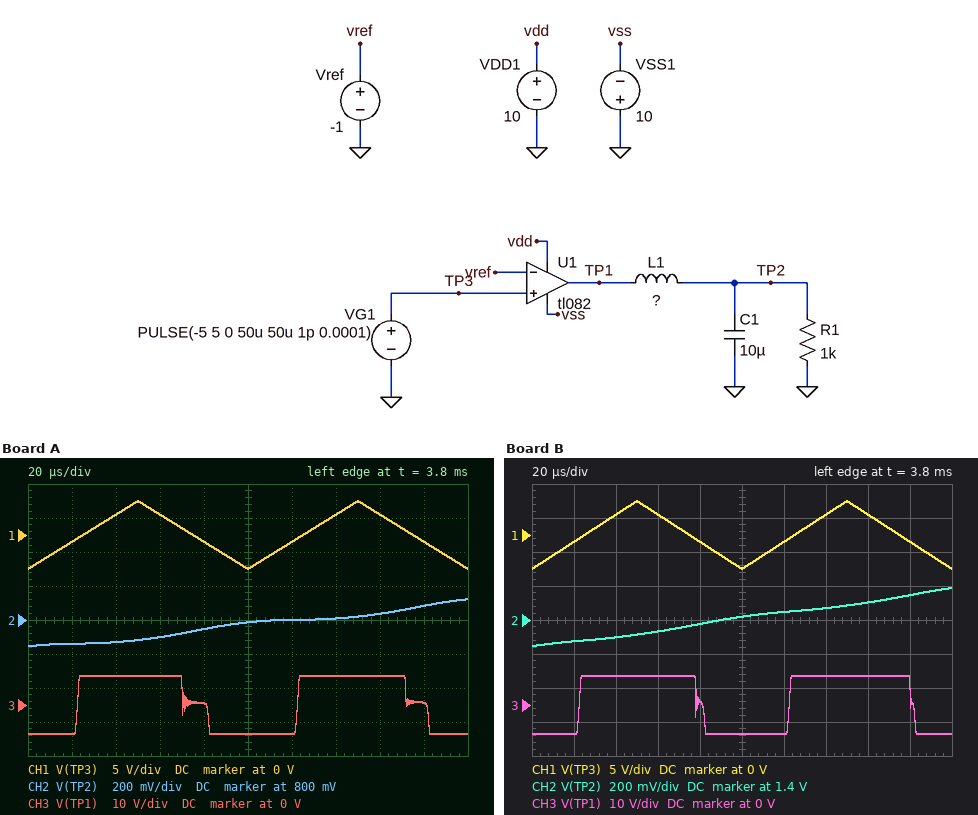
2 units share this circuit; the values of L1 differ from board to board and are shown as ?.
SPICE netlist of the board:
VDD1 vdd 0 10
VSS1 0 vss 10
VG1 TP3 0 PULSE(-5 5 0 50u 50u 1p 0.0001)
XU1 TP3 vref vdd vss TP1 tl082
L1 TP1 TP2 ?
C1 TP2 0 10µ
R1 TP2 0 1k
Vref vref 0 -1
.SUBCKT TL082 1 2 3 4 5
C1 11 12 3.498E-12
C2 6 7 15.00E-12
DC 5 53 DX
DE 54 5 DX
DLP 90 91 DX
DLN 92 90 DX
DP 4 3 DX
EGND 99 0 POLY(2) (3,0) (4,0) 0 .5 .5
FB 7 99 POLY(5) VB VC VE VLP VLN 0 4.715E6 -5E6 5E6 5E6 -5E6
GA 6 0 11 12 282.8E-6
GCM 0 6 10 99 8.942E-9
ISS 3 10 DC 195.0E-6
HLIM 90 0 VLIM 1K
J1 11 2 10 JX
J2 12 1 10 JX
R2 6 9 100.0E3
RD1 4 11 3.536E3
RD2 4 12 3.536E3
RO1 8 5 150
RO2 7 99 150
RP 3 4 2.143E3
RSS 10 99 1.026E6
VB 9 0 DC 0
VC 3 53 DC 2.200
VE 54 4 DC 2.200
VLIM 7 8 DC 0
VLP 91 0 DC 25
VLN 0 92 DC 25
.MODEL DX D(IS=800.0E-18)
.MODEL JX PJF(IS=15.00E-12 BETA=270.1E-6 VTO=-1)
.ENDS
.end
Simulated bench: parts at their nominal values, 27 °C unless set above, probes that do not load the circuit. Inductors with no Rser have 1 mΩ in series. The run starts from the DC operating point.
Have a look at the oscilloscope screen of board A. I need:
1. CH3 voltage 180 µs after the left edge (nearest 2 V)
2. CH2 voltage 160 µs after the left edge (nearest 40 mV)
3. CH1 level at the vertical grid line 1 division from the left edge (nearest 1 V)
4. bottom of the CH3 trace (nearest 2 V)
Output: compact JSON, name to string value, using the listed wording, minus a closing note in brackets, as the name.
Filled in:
{"CH3 voltage 180 µs after the left edge": "0 V", "CH2 voltage 160 µs after the left edge": "840 mV", "CH1 level at the vertical grid line 1 division from the left edge": "-1 V", "bottom of the CH3 trace": "-8 V"}
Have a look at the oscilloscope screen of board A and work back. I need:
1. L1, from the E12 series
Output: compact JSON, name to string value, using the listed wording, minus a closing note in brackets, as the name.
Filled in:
{"L1, from the E12 series": "15 mH"}
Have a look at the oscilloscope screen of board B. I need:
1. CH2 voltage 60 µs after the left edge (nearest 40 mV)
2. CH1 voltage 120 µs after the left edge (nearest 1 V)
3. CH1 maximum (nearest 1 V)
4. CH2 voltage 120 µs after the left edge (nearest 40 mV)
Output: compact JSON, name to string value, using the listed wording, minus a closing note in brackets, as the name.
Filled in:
{"CH2 voltage 60 µs after the left edge": "1.32 V", "CH1 voltage 120 µs after the left edge": "-1 V", "CH1 maximum": "5 V", "CH2 voltage 120 µs after the left edge": "1.44 V"}
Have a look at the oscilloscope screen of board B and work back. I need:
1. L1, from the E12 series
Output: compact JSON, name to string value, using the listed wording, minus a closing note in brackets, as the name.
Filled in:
{"L1, from the E12 series": "27 mH"}
